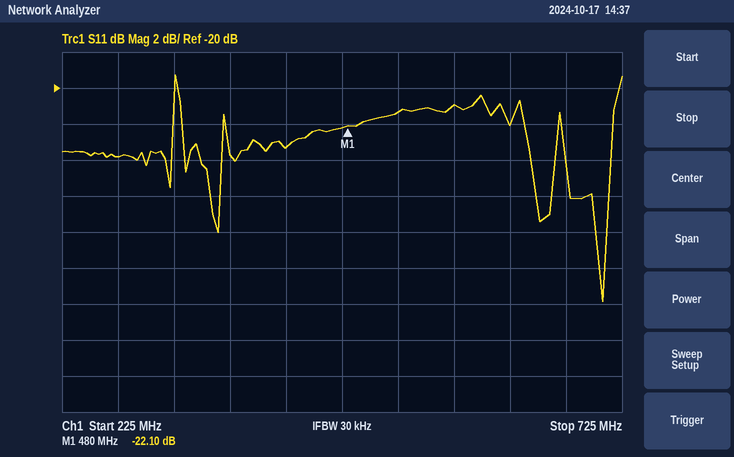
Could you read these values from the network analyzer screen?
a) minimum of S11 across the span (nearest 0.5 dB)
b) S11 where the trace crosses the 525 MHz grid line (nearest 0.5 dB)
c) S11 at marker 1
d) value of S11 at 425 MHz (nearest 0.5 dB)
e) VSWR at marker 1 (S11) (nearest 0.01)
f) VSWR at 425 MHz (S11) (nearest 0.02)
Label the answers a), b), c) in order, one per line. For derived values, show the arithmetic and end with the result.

a) -32.0 dB
b) -21.5 dB
c) -22.10 dB
d) -23.5 dB
e) (1 + 0.0785)/(1 − 0.0785) ≈ 1.17
f) |Γ| = 10^(-23.5/20) = 0.0668; VSWR = (1 + 0.0668)/(1 − 0.0668) ≈ 1.14
